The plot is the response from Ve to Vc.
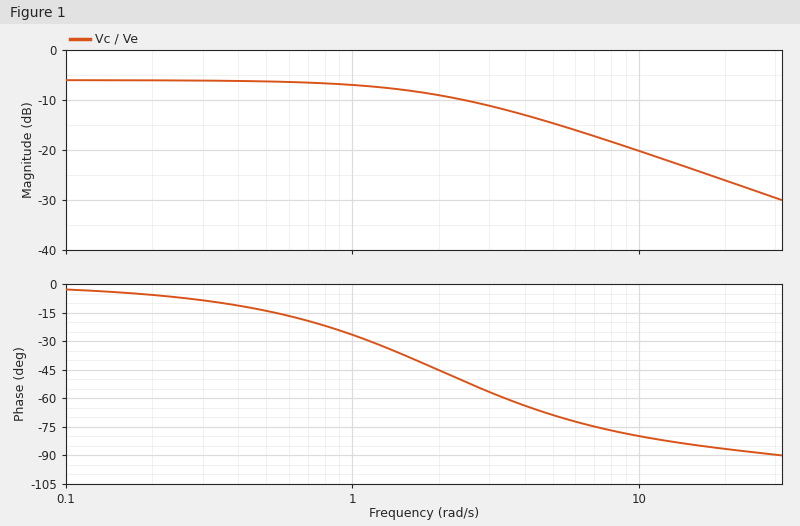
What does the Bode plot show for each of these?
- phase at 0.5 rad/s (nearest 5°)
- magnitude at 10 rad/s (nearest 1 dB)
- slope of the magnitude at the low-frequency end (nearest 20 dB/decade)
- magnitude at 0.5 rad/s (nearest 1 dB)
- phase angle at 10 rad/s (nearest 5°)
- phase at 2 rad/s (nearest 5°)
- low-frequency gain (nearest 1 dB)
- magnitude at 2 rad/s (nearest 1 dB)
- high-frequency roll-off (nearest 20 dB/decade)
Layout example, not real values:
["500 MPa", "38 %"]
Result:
["-15°", "-20 dB", "0 dB/decade", "-6 dB", "-80°", "-45°", "-6 dB", "-9 dB", "-20 dB/decade"]
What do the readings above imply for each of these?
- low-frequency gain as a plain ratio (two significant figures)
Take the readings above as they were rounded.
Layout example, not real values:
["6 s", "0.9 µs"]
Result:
["0.50"]
